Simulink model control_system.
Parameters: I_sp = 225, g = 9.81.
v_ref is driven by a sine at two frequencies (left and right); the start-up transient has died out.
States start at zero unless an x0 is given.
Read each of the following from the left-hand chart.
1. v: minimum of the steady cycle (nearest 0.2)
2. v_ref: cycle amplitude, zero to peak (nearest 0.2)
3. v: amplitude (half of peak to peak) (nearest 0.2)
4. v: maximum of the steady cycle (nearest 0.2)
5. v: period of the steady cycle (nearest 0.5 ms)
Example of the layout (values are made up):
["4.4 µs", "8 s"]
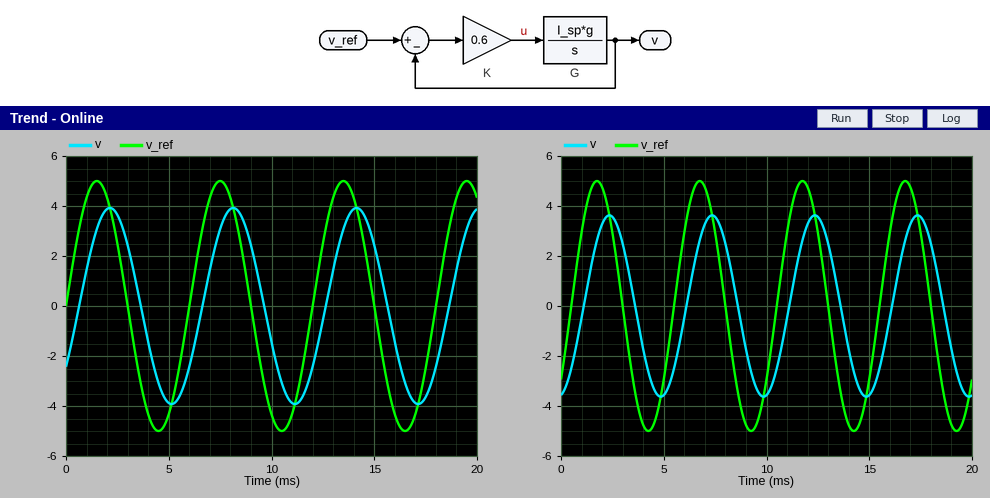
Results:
["-4.0", "5.0", "4.0", "4.0", "6.0 ms"]
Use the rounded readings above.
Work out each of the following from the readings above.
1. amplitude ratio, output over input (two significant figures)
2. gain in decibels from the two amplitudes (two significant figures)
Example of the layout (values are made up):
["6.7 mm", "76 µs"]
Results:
["0.80", "-1.9 dB"]
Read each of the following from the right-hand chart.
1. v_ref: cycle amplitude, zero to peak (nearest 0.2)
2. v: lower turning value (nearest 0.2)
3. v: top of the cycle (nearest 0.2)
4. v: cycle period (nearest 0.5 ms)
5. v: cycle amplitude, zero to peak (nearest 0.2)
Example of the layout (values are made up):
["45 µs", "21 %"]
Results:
["5.0", "-3.6", "3.6", "5.0 ms", "3.6"]
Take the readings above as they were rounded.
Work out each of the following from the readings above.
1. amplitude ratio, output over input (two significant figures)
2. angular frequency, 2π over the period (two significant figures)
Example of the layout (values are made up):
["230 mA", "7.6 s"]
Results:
["0.72", "1.3 rad/ms"]
